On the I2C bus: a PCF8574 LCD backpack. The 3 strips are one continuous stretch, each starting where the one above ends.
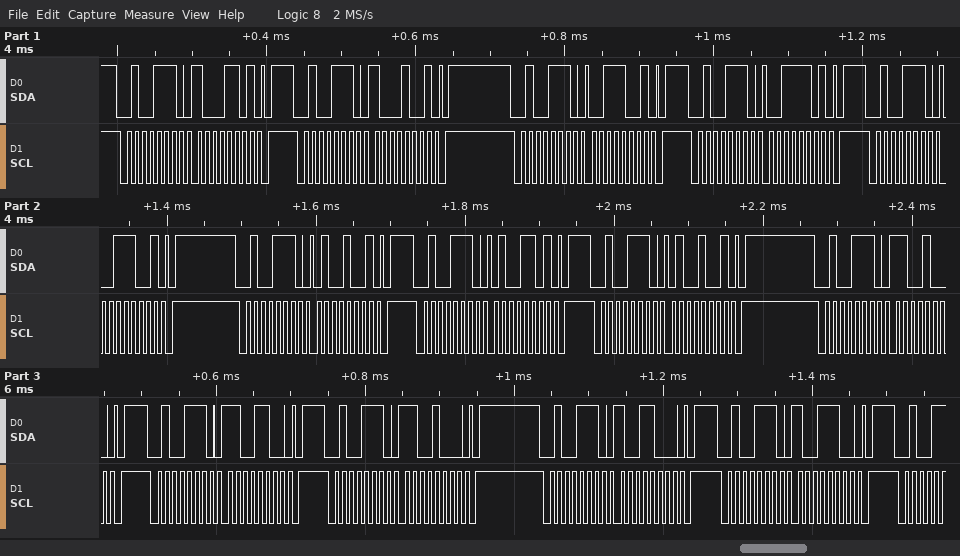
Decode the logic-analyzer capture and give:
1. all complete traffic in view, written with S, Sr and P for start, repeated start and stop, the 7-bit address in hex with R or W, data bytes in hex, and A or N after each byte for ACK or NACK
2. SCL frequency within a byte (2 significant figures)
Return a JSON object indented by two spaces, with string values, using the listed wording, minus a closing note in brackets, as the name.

{
  "all complete traffic in view, written with S, Sr and P for start, repeated start and stop, the 7-bit address in hex with R or W, data bytes in hex, and A or N after each byte for ACK or NACK": "S 27W A 8D A P S 27W A 89 A P S 27W A 39 A P S 27W A 3D A P S 27W A 39 A P S 27W A 49 A P S 27W A 4D A P S 27W A 49 A P S 27W A C8 A P S 27W A CC A P S 27W A C8 A P S 27W A 98 A P S 27W A 9C A P",
  "SCL frequency within a byte": "100 kHz"
}
